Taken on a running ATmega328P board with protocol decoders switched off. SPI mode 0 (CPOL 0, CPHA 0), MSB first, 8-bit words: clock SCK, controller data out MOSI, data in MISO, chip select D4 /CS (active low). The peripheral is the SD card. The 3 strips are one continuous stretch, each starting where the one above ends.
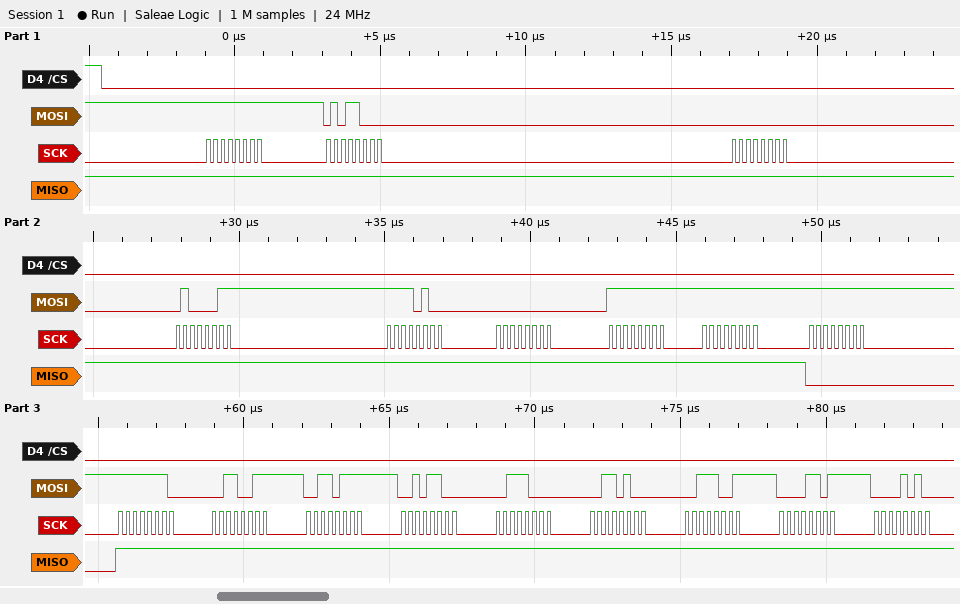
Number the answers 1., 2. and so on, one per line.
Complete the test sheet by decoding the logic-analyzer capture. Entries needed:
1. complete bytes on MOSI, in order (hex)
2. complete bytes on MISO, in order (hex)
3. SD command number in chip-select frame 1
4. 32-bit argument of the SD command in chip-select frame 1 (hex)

1. FF 58 00 43 F4 00 FF FF FF FE 33 37 2C 38 34 39 0D 0A
2. FF FF FF FF FF FF FF FF 00 FF FF FF FF FF FF FF FF FF
3. CMD24
4. 0x0043F400
